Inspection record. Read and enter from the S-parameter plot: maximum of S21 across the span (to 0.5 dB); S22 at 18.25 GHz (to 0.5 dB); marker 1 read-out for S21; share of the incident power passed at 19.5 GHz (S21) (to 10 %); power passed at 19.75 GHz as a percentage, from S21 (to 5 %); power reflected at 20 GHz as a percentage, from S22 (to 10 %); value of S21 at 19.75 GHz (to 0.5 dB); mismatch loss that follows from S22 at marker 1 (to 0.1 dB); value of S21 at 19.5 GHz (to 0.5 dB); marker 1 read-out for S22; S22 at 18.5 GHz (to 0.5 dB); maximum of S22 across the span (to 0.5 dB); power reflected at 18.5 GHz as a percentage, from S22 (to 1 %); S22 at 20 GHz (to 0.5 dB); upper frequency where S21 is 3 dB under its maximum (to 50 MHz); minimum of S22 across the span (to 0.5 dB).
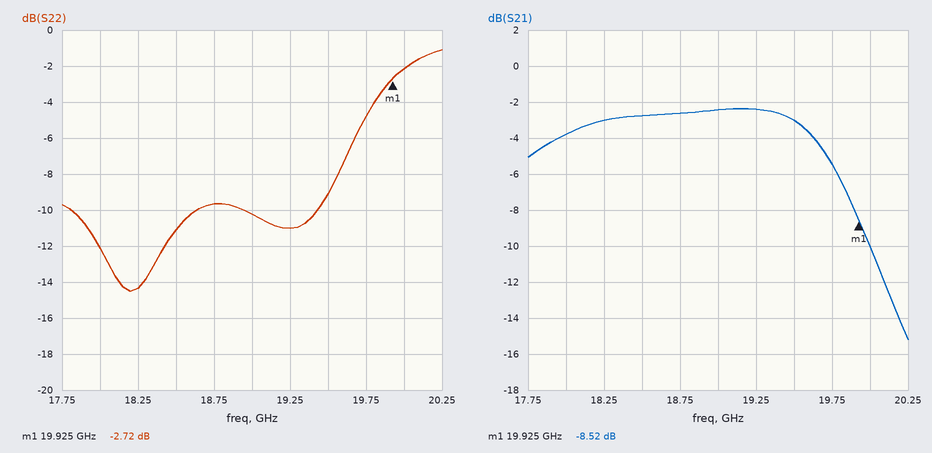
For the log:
-2.5 dB
-14.5 dB
-8.52 dB
50 %
30 %
60 %
-5.5 dB
3.3 dB
-3.0 dB
-2.72 dB
-11.0 dB
-1.0 dB
8 %
-2.0 dB
19.75 GHz
-14.5 dB
